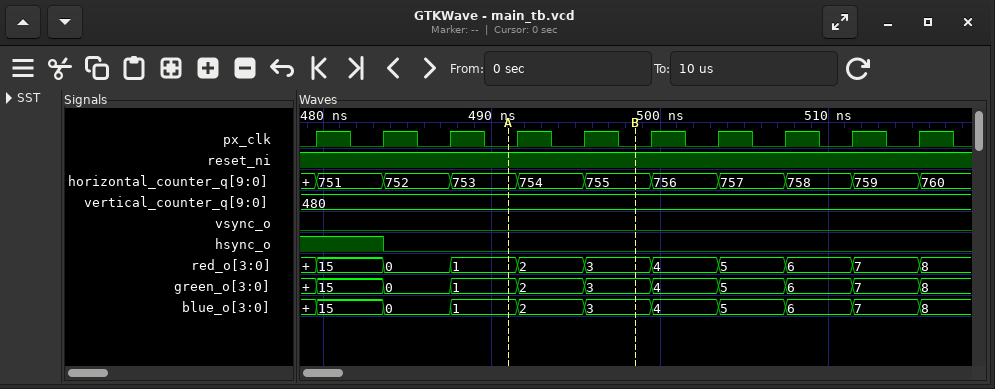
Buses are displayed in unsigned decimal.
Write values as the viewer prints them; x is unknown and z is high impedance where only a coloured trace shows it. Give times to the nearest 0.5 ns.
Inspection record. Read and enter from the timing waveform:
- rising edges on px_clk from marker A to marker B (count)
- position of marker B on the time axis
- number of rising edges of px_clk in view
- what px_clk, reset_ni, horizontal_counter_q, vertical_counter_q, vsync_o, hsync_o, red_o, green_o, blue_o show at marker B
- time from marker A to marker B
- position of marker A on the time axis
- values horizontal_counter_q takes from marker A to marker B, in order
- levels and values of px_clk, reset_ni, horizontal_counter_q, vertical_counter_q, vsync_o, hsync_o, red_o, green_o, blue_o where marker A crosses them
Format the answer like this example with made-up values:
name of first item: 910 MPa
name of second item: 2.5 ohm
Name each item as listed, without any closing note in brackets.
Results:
rising edges on px_clk from marker A to marker B: 2
position of marker B on the time axis: 498.5 ns
number of rising edges of px_clk in view: 10
what px_clk, reset_ni, horizontal_counter_q, vertical_counter_q, vsync_o, hsync_o, red_o, green_o, blue_o show at marker B: px_clk=0, reset_ni=1, horizontal_counter_q=755, vertical_counter_q=480, vsync_o=0, hsync_o=0, red_o=3, green_o=3, blue_o=3
time from marker A to marker B: 7.5 ns
position of marker A on the time axis: 491 ns
values horizontal_counter_q takes from marker A to marker B, in order: 753, 754, 755
levels and values of px_clk, reset_ni, horizontal_counter_q, vertical_counter_q, vsync_o, hsync_o, red_o, green_o, blue_o where marker A crosses them: px_clk=0, reset_ni=1, horizontal_counter_q=753, vertical_counter_q=480, vsync_o=0, hsync_o=0, red_o=1, green_o=1, blue_o=1
